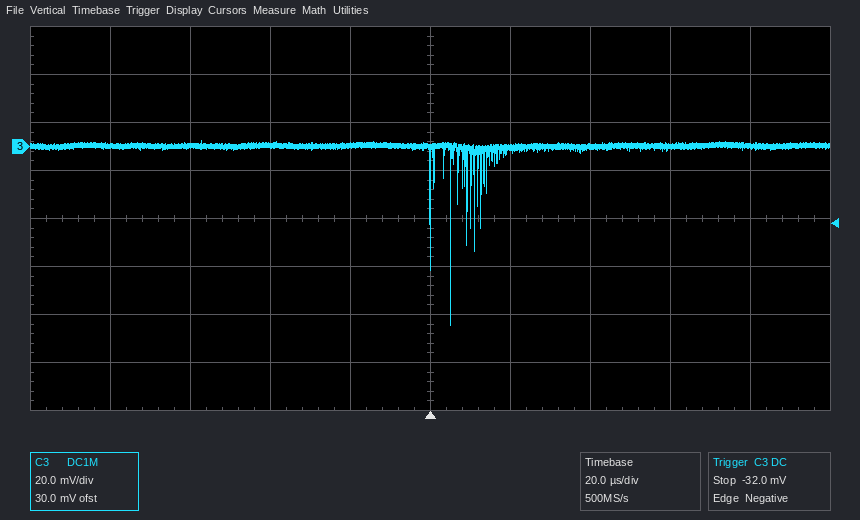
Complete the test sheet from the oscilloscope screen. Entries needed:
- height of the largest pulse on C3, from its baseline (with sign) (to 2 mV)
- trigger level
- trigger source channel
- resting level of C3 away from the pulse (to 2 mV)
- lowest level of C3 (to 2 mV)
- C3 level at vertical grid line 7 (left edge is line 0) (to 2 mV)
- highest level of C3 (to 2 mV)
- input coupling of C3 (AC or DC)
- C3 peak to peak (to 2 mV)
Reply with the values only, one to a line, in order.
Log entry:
-74 mV
-32.0 mV
C3
0 mV
-74 mV
0 mV
2 mV
DC
76 mV
